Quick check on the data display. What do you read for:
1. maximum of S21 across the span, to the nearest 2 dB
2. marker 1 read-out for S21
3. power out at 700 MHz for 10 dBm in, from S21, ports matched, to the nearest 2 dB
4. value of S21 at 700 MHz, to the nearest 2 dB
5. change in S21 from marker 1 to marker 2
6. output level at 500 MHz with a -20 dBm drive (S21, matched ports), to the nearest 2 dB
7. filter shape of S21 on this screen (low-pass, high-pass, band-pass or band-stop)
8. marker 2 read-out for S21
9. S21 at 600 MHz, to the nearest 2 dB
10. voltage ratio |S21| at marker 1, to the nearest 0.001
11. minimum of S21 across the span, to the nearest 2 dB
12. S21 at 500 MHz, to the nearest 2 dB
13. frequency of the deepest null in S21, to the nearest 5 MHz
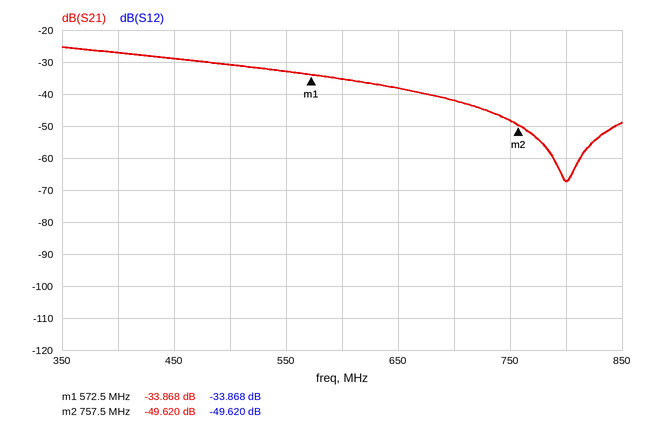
-26 dB
-33.868 dB
-32 dBm
-42 dB
-15.752 dB
-50 dBm
low-pass
-49.620 dB
-36 dB
0.020
-68 dB
-30 dB
800 MHz
